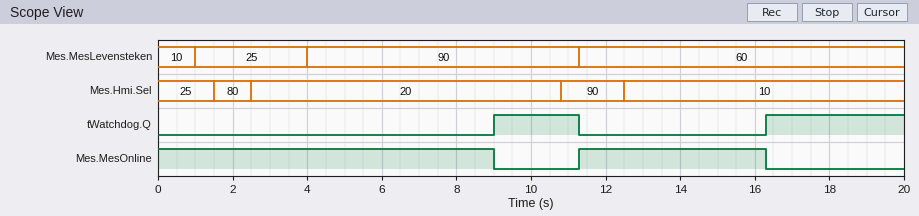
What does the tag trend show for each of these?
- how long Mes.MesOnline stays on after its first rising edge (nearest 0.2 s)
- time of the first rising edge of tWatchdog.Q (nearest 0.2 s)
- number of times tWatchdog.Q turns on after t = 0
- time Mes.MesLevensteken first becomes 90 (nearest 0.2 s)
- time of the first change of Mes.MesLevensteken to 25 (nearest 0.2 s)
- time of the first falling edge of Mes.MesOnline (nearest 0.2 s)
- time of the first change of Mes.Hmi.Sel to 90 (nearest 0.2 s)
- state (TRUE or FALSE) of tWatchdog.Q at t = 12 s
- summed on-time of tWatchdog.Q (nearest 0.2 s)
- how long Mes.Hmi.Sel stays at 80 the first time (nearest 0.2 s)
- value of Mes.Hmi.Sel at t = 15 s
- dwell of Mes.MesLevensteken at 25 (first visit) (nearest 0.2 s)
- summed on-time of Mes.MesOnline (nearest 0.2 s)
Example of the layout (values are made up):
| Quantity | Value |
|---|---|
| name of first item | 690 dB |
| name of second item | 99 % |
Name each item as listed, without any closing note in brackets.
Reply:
| Quantity | Value |
|---|---|
| how long Mes.MesOnline stays on after its first rising edge | 5.0 s |
| time of the first rising edge of tWatchdog.Q | 9.0 s |
| number of times tWatchdog.Q turns on after t = 0 | 2 |
| time Mes.MesLevensteken first becomes 90 | 4.0 s |
| time of the first change of Mes.MesLevensteken to 25 | 1.0 s |
| time of the first falling edge of Mes.MesOnline | 9.0 s |
| time of the first change of Mes.Hmi.Sel to 90 | 10.8 s |
| state (TRUE or FALSE) of tWatchdog.Q at t = 12 s | FALSE |
| summed on-time of tWatchdog.Q | 6.0 s |
| how long Mes.Hmi.Sel stays at 80 the first time | 1.0 s |
| value of Mes.Hmi.Sel at t = 15 s | 10 |
| dwell of Mes.MesLevensteken at 25 (first visit) | 3.0 s |
| summed on-time of Mes.MesOnline | 14.0 s |
